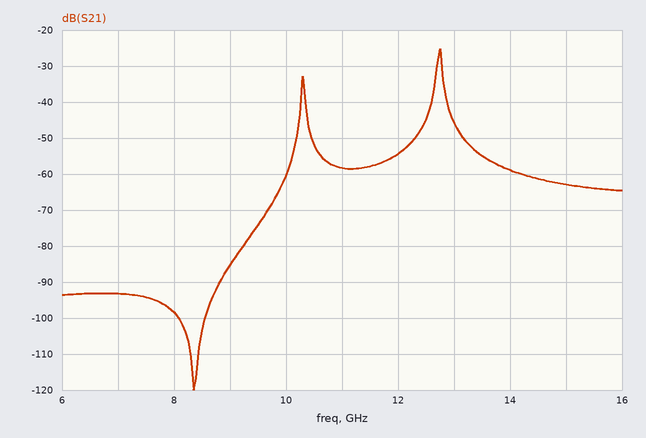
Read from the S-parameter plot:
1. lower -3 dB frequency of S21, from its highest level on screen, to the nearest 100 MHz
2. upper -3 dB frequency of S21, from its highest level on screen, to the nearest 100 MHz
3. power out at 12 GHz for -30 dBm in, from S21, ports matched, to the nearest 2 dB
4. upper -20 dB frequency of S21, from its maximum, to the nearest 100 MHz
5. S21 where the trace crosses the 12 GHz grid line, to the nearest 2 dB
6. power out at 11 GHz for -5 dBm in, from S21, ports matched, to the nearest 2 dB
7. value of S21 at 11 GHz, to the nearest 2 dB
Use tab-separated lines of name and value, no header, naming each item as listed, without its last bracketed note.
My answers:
lower -3 dB frequency of S21, from its highest level on screen, to the nearest 100 MHz	12.7 GHz
upper -3 dB frequency of S21, from its highest level on screen, to the nearest 100 MHz	12.8 GHz
power out at 12 GHz for -30 dBm in, from S21, ports matched, to the nearest 2 dB	-84 dBm
upper -20 dB frequency of S21, from its maximum, to the nearest 100 MHz	13.0 GHz
S21 where the trace crosses the 12 GHz grid line, to the nearest 2 dB	-54 dB
power out at 11 GHz for -5 dBm in, from S21, ports matched, to the nearest 2 dB	-64 dBm
value of S21 at 11 GHz, to the nearest 2 dB	-58 dB
